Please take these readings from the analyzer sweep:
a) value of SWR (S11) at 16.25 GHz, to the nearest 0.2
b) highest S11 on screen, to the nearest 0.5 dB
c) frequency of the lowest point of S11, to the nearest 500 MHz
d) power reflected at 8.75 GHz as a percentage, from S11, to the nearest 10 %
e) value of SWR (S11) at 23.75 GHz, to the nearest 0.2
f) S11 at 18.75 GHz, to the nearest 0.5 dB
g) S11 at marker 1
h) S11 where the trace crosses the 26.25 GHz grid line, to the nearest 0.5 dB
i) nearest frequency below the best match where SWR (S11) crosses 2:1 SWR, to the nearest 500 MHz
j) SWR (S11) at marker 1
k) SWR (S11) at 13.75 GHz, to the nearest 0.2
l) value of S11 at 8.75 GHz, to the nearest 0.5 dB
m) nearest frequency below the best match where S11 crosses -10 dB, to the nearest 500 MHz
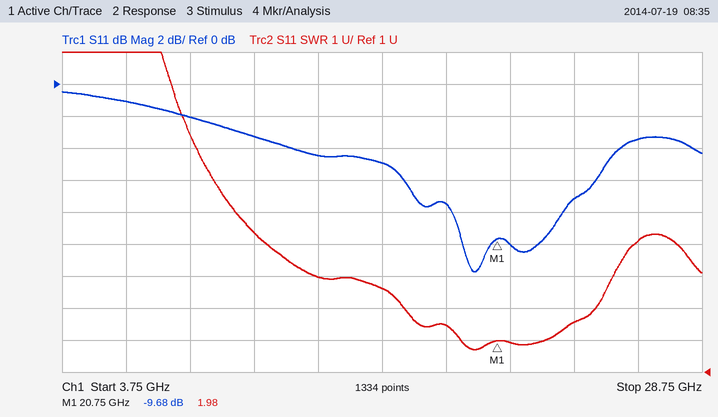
3.6
-0.5 dB
20.0 GHz
60 %
2.6
-7.5 dB
-9.68 dB
-3.5 dB
19.5 GHz
1.98
4.0
-2.0 dB
19.5 GHz
